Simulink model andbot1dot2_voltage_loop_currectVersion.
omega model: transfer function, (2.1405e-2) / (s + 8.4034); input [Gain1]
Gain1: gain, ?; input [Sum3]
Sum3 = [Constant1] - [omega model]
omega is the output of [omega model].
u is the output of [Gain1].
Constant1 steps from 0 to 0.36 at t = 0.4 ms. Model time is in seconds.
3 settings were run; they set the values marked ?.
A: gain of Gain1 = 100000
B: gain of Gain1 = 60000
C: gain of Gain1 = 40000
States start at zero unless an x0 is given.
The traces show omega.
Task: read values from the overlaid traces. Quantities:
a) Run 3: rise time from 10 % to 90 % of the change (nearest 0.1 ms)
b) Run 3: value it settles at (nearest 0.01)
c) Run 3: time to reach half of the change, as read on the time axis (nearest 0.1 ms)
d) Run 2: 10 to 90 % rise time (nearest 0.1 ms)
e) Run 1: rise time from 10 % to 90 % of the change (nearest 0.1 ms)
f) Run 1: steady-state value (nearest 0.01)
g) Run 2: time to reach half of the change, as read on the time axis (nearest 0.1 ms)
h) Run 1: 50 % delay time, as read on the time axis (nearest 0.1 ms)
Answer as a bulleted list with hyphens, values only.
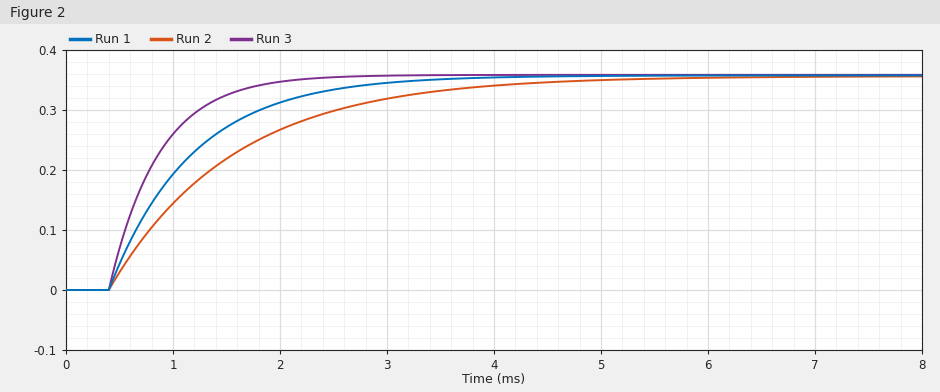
- 1.0 ms
- 0.36
- 0.7 ms
- 2.5 ms
- 1.7 ms
- 0.36
- 1.2 ms
- 0.9 ms
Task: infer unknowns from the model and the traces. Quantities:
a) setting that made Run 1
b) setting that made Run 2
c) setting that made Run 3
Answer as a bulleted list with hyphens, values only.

- B
- C
- A
